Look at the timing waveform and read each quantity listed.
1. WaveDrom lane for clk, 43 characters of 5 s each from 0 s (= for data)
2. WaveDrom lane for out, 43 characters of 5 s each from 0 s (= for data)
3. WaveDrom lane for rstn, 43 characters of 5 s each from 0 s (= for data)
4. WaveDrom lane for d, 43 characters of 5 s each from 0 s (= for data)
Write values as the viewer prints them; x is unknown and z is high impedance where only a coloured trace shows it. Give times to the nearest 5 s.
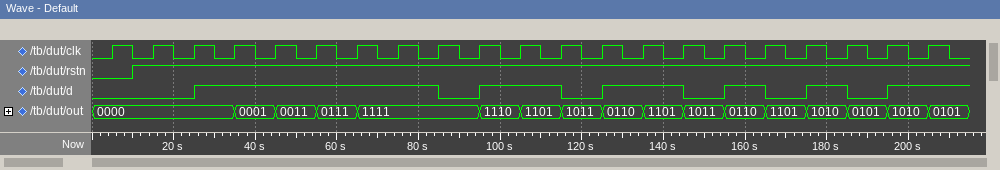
{name: 'clk', wave: '0101010101010101010101010101010101010101010'}
{name: 'out', wave: '=......=.=.=.=.....=.=.=.=.=.=.=.=.=.=.=.=.', data: '0000 0001 0011 0111 1111 1110 1101 1011 0110 1101 1011 0110 1101 1010 0101 1010 0101'}
{name: 'rstn', wave: '0.1........................................'}
{name: 'd', wave: '0....1...........0.1...0.1...0.1.0.1.0.1...'}
